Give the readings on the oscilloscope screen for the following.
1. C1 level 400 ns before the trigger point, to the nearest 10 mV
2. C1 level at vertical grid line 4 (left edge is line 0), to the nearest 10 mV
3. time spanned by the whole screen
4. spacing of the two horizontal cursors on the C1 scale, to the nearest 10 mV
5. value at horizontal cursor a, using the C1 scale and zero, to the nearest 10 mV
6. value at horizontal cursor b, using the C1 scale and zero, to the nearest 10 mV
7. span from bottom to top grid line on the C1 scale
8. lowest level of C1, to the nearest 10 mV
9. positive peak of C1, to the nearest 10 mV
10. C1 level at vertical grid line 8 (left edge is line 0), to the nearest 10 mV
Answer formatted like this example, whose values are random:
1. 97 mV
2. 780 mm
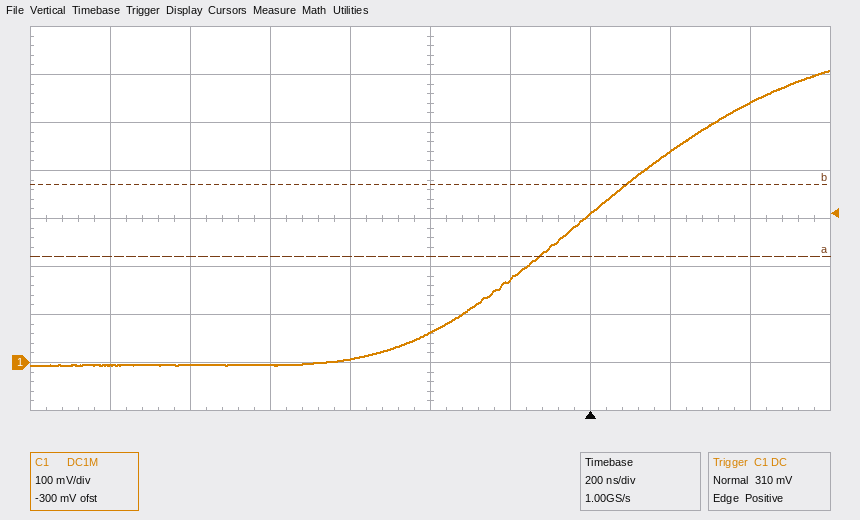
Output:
1. 60 mV
2. 10 mV
3. 2 µs
4. 150 mV
5. 220 mV
6. 370 mV
7. 800 mV
8. -10 mV
9. 610 mV
10. 440 mV
